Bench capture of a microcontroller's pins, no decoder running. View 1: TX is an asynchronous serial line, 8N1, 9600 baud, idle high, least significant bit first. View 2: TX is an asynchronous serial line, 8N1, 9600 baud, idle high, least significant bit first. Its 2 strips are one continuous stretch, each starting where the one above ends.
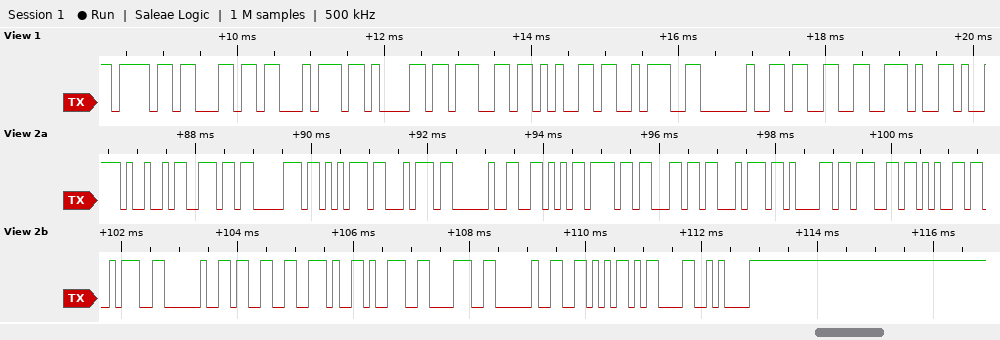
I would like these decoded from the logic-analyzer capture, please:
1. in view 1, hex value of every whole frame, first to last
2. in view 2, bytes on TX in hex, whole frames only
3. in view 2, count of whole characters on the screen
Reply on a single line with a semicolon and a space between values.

6F 6C 74 61 67 65 3A 20 33 2E; 0x49 0x6E 0x70 0x75 0x74 0x20 0x56 0x6F 0x6C 0x74 0x61 0x67 0x65 0x3A 0x20 0x33 0x2E 0x39 0x38 0x20 0x56 0x0D 0x0A; 23
